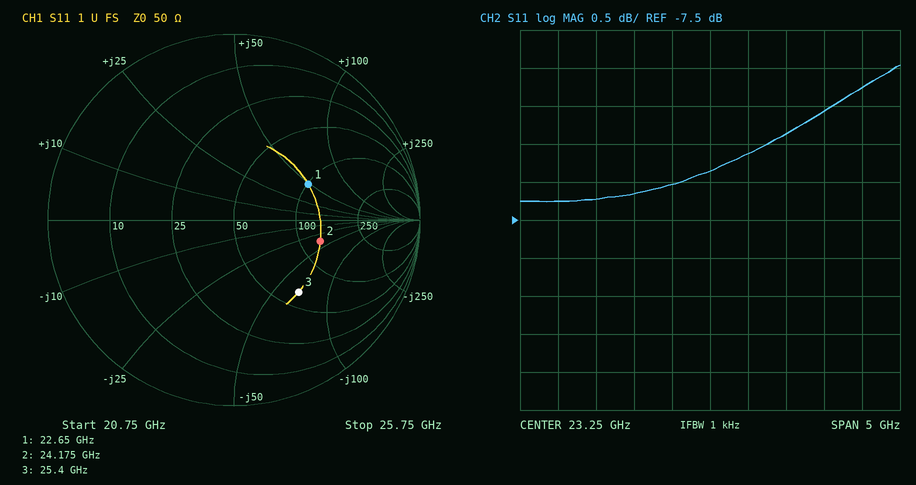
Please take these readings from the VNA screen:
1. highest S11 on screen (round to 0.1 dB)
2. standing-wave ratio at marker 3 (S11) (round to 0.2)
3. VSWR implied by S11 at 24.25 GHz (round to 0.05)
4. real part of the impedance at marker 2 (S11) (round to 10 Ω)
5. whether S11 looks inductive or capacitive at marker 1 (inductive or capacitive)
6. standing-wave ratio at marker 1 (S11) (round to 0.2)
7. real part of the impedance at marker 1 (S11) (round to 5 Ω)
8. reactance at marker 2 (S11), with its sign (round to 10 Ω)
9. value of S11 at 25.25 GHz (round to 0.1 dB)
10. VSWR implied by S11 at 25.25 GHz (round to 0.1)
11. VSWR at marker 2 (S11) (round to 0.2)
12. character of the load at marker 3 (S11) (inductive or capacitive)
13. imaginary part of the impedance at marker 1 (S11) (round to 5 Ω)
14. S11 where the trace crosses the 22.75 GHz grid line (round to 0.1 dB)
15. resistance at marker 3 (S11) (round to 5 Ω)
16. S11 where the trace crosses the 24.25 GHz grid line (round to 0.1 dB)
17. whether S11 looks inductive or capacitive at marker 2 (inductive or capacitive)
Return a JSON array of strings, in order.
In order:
["-5.5 dB", "3.2", "2.85", "130 Ω", "inductive", "2.6", "100 Ω", "-40 Ω", "-5.8 dB", "3.1", "2.8", "capacitive", "+50 Ω", "-7.0 dB", "65 Ω", "-6.4 dB", "capacitive"]
